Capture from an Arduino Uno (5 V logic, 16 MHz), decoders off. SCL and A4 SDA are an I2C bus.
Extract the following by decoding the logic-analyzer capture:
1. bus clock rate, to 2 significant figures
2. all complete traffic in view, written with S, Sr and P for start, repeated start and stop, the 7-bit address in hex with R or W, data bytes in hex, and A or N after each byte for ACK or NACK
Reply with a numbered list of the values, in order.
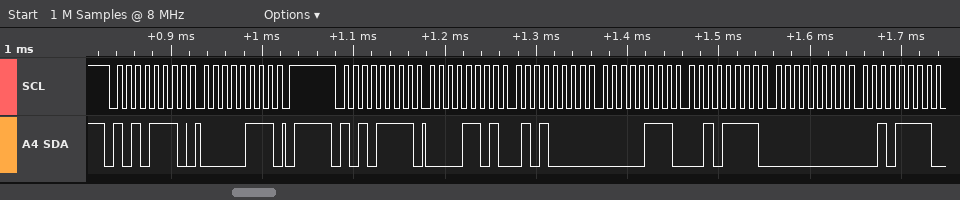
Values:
1. 100 kHz
2. S 57W A 07 A P S 57R A 0D A 50 A 07 A 2F A 00 A 2F A
